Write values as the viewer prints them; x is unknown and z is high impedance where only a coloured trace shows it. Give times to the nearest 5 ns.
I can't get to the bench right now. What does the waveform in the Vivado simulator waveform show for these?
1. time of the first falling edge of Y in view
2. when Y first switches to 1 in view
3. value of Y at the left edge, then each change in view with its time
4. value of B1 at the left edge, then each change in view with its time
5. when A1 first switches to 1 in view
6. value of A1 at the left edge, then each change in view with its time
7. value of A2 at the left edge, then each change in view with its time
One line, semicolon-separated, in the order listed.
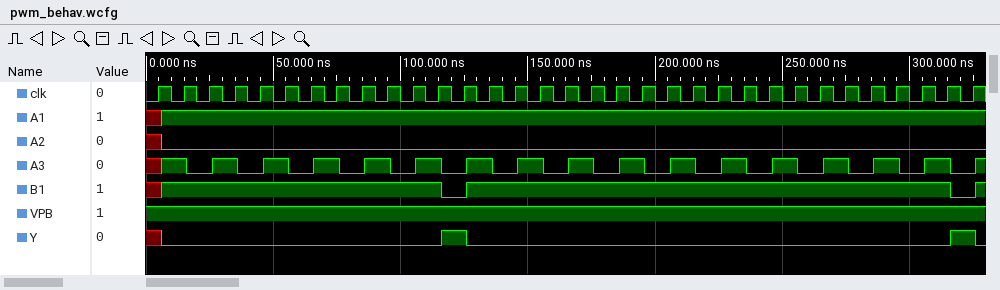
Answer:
125 ns; 115 ns; x, 0 at 5 ns, 1 at 115 ns, 0 at 125 ns, 1 at 315 ns, 0 at 325 ns; x, 1 at 5 ns, 0 at 115 ns, 1 at 125 ns, 0 at 315 ns, 1 at 325 ns; 5 ns; x, 1 at 5 ns; x, 0 at 5 ns
